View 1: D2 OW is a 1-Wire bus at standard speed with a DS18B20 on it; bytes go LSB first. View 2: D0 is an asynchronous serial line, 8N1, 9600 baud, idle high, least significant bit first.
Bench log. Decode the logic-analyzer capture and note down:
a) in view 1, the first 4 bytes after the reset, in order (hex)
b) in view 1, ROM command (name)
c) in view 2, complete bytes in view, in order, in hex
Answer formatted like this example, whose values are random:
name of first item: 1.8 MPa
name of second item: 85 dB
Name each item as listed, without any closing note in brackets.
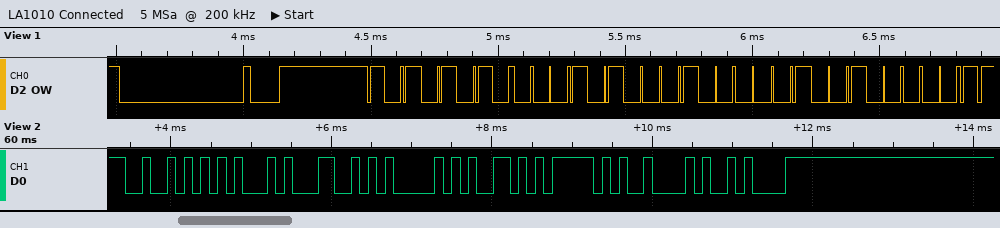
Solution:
in view 1, the first 4 bytes after the reset, in order: 55 28 82 04
in view 1, ROM command: Match ROM
in view 2, complete bytes in view, in order, in hex: 52 45 4C 41 59 5F 42 0A
